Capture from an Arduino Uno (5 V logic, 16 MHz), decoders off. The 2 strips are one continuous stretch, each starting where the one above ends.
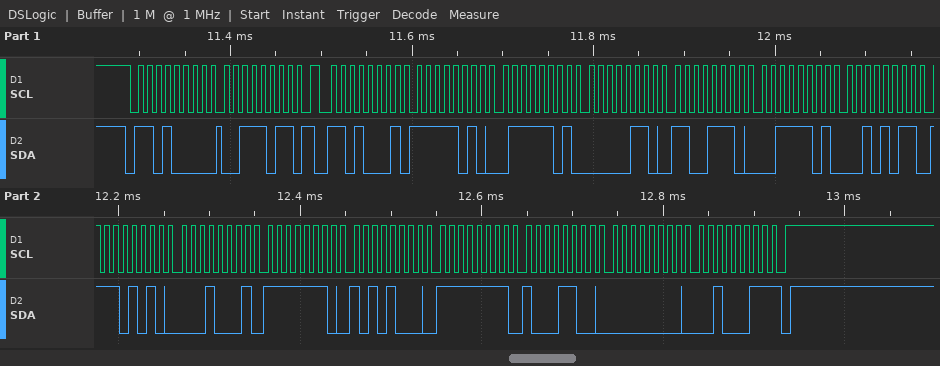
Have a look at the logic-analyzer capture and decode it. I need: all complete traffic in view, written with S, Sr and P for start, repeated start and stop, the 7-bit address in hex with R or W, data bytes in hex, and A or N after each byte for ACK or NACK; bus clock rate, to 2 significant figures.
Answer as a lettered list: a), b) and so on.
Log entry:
a) S 68W A 3B A Sr 68R A FA A 7D A 06 A CE A 3D A 2B A EA A 11 A FE A A8 A FF A 8C A 00 A 23 N P
b) 100 kHz
